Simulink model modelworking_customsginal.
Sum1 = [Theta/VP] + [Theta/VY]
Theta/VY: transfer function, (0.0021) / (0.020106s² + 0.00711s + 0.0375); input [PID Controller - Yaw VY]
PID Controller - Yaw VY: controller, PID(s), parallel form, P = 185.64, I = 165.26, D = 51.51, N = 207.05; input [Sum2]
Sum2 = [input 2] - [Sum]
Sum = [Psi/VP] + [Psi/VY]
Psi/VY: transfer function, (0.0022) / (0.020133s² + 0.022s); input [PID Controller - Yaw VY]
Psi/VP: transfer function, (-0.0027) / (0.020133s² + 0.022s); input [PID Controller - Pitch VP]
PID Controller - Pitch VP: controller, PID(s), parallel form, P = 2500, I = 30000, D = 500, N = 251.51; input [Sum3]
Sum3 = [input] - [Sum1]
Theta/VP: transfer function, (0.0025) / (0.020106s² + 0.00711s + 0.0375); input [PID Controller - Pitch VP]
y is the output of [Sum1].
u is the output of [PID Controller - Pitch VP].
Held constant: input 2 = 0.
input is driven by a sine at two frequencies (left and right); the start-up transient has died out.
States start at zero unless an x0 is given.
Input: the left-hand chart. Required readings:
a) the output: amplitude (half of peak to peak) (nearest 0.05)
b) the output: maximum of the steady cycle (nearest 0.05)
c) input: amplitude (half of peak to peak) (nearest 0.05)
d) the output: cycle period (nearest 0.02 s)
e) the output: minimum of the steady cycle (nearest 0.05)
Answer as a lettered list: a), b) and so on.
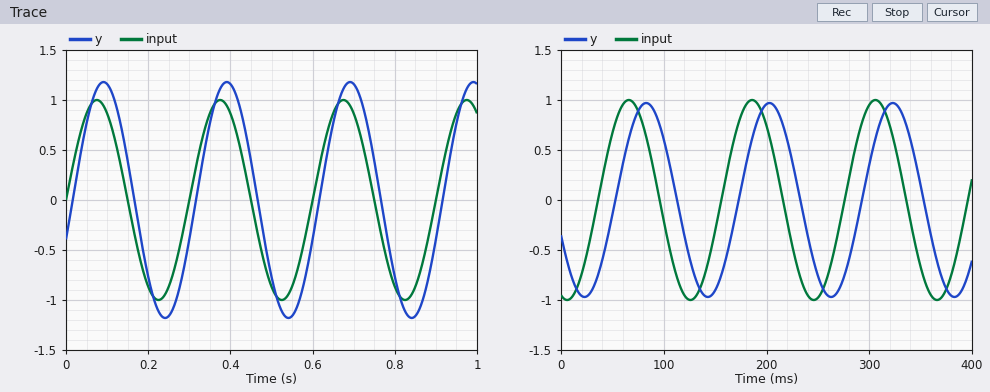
a) 1.20
b) 1.20
c) 1.00
d) 0.30 s
e) -1.20
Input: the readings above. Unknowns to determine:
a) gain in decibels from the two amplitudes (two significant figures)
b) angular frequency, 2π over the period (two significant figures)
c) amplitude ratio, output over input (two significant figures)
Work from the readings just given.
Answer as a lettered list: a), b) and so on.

a) 1.6 dB
b) 21 rad/s
c) 1.2
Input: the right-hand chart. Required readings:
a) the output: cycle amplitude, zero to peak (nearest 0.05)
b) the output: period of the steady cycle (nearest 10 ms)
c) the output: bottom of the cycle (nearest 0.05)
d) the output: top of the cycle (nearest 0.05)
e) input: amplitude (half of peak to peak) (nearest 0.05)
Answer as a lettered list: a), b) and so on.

a) 0.95
b) 120 ms
c) -0.95
d) 0.95
e) 1.00
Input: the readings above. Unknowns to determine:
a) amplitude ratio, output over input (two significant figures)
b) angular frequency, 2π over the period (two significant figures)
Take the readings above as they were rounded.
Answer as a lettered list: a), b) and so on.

a) 0.95
b) 0.052 rad/ms
